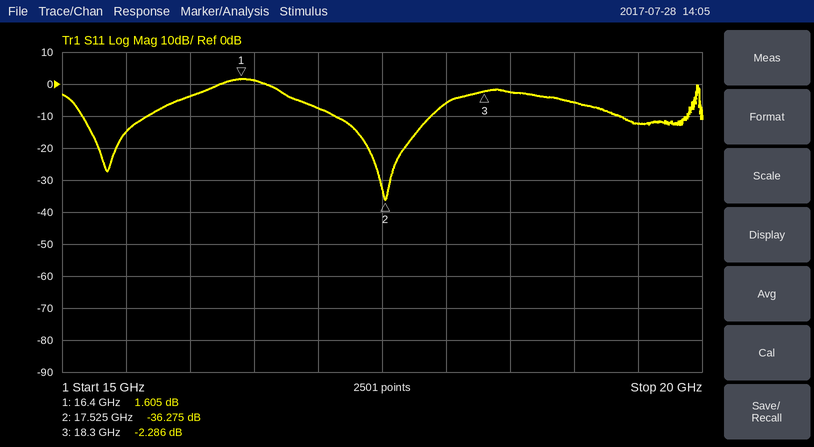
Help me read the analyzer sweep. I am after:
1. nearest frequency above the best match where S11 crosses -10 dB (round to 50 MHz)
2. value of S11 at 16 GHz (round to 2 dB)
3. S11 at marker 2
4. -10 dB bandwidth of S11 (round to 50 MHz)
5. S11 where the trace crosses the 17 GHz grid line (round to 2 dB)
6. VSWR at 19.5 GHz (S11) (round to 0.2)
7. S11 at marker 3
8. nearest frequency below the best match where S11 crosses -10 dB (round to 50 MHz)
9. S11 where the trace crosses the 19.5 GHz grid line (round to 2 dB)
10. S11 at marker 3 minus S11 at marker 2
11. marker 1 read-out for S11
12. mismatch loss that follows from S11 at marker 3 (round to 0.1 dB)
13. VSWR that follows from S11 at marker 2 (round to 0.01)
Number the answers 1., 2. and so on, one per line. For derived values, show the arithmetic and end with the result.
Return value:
1. 17.90 GHz
2. -4 dB
3. -36.275 dB
4. 17.90 GHz − 17.15 GHz = 750 MHz
5. -8 dB
6. |Γ| = 10^(-12/20) = 0.2512; VSWR = (1 + 0.2512)/(1 − 0.2512) ≈ 1.67, so 1.6 to the nearest 0.2
7. -2.286 dB
8. 17.15 GHz
9. -12 dB
10. -2.286 − (-36.275) = 33.989 dB
11. 1.605 dB
12. −10 log10(1 − 10^(-2.286/10)) ≈ 3.9 dB
13. (1 + 0.0154)/(1 − 0.0154) ≈ 1.03
